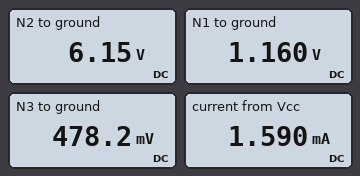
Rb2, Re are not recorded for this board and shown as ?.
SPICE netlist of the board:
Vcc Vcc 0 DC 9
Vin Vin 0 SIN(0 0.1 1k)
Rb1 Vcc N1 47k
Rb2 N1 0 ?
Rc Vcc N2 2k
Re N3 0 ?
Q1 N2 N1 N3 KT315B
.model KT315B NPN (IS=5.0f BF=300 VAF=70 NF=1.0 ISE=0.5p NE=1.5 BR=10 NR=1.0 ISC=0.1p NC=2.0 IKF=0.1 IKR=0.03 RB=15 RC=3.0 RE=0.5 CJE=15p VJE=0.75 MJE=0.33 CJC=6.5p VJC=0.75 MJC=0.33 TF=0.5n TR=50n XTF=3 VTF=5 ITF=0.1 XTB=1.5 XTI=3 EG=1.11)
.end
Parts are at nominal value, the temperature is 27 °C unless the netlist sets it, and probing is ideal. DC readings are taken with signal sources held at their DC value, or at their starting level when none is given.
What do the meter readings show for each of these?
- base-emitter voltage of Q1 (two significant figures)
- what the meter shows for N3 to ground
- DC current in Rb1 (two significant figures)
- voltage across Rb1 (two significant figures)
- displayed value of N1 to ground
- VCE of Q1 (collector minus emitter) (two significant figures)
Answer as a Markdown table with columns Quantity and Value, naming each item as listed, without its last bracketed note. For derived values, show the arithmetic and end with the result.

| Quantity | Value |
|---|---|
| base-emitter voltage of Q1 | 1.16 V - 478.2 mV = 680 mV |
| what the meter shows for N3 to ground | 478.2 mV |
| DC current in Rb1 | (9 V - 1.16 V) / 47 kΩ = 170 µA |
| voltage across Rb1 | 9 V - 1.16 V = 7.8 V |
| displayed value of N1 to ground | 1.160 V |
| VCE of Q1 (collector minus emitter) | 6.15 V - 478.2 mV = 5.7 V |
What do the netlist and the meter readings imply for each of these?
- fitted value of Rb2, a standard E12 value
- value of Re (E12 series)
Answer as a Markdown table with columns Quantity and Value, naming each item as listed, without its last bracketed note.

| Quantity | Value |
|---|---|
| fitted value of Rb2, a standard E12 value | 8.2 kΩ |
| value of Re | 330 Ω |
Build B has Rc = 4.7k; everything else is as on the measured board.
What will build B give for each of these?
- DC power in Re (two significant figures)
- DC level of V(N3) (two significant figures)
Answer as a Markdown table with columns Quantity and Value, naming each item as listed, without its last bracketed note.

| Quantity | Value |
|---|---|
| DC power in Re | 680 µW |
| DC level of V(N3) | 470 mV |
